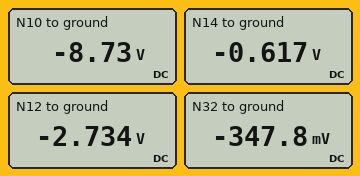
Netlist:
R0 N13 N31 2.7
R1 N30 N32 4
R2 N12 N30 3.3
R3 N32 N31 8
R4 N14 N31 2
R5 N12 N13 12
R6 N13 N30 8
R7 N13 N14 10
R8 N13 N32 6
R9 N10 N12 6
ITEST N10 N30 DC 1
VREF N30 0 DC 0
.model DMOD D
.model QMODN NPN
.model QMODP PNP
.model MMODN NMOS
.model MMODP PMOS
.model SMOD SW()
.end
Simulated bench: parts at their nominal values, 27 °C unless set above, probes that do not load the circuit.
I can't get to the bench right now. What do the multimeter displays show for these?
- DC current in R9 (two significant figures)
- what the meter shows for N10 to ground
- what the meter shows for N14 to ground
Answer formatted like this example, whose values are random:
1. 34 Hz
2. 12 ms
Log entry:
1. 1.0 A
2. -8.73 V
3. -0.617 V
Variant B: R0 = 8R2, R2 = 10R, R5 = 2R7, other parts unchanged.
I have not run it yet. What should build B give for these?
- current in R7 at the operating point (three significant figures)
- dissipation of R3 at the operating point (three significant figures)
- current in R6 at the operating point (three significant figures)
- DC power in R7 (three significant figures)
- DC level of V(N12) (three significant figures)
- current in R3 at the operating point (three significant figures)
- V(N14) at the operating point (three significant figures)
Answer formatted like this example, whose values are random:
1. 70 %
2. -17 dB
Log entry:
1. 38.4 mA
2. 71.5 mW
3. 301 mA
4. 14.7 mW
5. -4.02 V
6. 94.5 mA
7. -2.02 V
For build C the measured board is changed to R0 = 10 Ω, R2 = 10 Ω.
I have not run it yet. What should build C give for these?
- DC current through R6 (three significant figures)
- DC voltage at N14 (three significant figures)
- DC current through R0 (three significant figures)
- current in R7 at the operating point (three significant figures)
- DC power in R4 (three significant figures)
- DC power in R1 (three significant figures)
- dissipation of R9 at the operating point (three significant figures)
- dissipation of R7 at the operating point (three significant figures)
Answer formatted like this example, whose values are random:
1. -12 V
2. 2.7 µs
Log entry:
1. 194 mA
2. -1.28 V
3. 32.0 mA
4. 26.7 mA
5. 1.42 mW
6. 145 mW
7. 6.00 W
8. 7.11 mW
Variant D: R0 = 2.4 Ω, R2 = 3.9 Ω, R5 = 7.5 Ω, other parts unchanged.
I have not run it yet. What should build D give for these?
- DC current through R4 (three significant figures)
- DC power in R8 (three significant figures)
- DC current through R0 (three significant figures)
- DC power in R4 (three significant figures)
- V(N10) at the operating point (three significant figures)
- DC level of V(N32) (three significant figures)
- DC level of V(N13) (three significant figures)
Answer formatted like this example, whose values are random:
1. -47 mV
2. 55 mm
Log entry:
1. 8.07 mA
2. 39.1 mW
3. 40.4 mA
4. 130 µW
5. -8.91 V
6. -517 mV
7. -1.00 V
